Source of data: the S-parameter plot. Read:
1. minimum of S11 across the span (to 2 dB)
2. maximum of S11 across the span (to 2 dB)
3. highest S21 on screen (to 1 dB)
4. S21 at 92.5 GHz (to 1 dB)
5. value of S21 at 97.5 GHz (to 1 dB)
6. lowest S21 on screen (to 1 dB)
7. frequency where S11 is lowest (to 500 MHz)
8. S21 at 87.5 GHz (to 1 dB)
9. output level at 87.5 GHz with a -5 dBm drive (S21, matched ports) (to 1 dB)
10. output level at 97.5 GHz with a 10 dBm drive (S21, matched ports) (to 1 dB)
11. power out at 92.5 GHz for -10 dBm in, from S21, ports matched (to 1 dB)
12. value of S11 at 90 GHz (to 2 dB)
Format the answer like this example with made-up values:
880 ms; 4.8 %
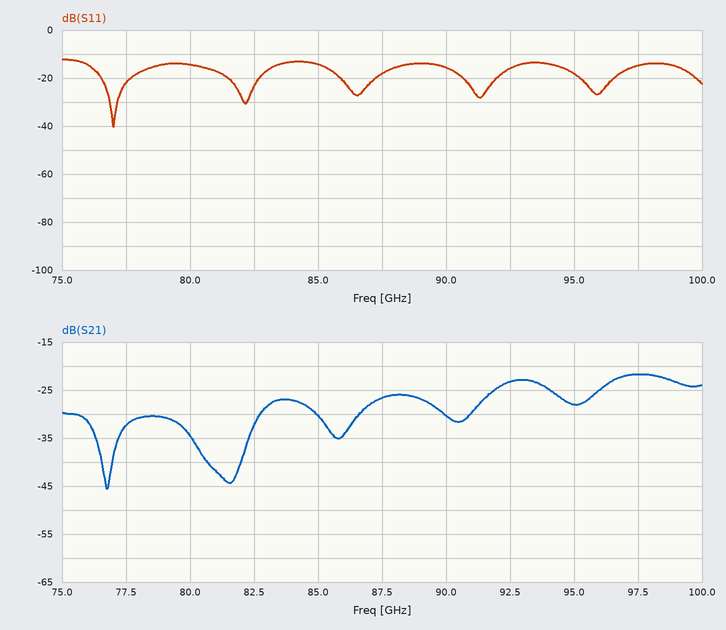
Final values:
-40 dB; -12 dB; -22 dB; -23 dB; -22 dB; -46 dB; 77.0 GHz; -27 dB; -32 dBm; -12 dBm; -33 dBm; -16 dB
